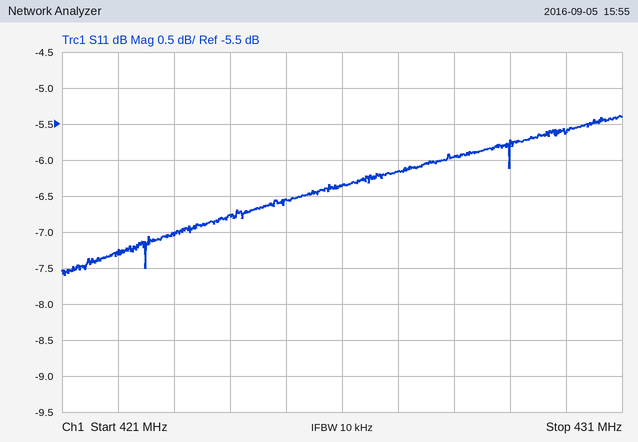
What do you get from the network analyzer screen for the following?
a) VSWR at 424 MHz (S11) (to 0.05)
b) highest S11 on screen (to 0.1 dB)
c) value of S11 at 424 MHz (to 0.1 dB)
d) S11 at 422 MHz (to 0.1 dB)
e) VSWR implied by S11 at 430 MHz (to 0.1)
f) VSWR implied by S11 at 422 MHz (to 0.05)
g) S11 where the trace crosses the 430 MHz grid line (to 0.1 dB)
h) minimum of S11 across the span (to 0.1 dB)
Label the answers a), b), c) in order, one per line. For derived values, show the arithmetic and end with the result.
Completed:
a) |Γ| = 10^(-6.8/20) = 0.4571; VSWR = (1 + 0.4571)/(1 − 0.4571) ≈ 2.68, so 2.70 to the nearest 0.05
b) -5.4 dB
c) -6.8 dB
d) -7.3 dB
e) |Γ| = 10^(-5.6/20) = 0.5248; VSWR = (1 + 0.5248)/(1 − 0.5248) ≈ 3.2
f) |Γ| = 10^(-7.3/20) = 0.4315; VSWR = (1 + 0.4315)/(1 − 0.4315) ≈ 2.52, so 2.50 to the nearest 0.05
g) -5.6 dB
h) -7.6 dB
